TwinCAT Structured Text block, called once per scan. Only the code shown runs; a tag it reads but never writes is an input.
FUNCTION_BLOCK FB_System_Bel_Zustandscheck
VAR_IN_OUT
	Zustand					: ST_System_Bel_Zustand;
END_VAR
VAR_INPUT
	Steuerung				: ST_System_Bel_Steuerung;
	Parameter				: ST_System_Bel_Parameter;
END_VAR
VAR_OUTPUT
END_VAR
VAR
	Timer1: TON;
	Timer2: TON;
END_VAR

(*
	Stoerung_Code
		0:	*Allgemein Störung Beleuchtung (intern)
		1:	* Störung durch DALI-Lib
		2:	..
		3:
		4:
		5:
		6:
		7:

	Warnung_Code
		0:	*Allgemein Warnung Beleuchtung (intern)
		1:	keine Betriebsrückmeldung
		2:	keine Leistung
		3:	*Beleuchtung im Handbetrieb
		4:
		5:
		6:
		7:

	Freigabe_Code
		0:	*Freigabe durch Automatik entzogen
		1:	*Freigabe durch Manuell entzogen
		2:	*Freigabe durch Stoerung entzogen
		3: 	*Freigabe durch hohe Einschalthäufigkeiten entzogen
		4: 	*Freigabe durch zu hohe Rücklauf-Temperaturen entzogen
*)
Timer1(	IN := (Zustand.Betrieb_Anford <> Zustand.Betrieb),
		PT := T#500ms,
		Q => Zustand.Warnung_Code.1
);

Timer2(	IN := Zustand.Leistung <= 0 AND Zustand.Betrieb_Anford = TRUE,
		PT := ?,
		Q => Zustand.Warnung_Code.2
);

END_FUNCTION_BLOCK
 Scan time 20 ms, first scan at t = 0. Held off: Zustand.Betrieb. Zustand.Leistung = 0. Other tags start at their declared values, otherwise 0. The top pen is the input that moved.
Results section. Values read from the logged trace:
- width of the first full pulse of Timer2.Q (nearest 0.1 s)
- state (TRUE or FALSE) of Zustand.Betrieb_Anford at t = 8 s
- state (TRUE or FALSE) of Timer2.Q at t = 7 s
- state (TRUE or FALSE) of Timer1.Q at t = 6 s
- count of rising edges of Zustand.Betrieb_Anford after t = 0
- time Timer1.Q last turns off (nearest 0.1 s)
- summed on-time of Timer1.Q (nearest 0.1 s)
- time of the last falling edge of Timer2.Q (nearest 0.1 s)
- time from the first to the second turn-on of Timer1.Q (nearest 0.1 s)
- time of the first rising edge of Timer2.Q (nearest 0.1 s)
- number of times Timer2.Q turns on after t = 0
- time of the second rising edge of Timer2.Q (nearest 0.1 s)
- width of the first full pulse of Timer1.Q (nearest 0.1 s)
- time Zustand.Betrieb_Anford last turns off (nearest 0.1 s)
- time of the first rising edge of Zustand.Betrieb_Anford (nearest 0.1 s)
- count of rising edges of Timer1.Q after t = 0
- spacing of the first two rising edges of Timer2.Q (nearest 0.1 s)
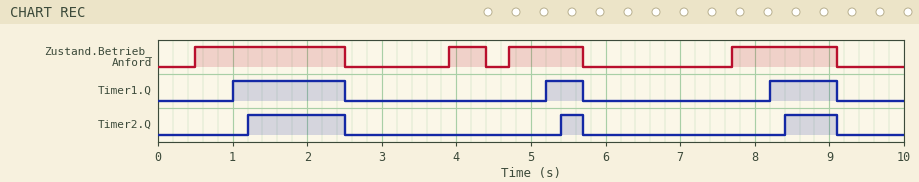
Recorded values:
1.3 s
TRUE
FALSE
FALSE
4
9.1 s
2.9 s
9.1 s
4.2 s
1.2 s
3
5.4 s
1.5 s
9.1 s
0.5 s
3
4.2 s
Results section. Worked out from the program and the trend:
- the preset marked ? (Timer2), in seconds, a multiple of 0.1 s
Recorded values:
0.7 s
